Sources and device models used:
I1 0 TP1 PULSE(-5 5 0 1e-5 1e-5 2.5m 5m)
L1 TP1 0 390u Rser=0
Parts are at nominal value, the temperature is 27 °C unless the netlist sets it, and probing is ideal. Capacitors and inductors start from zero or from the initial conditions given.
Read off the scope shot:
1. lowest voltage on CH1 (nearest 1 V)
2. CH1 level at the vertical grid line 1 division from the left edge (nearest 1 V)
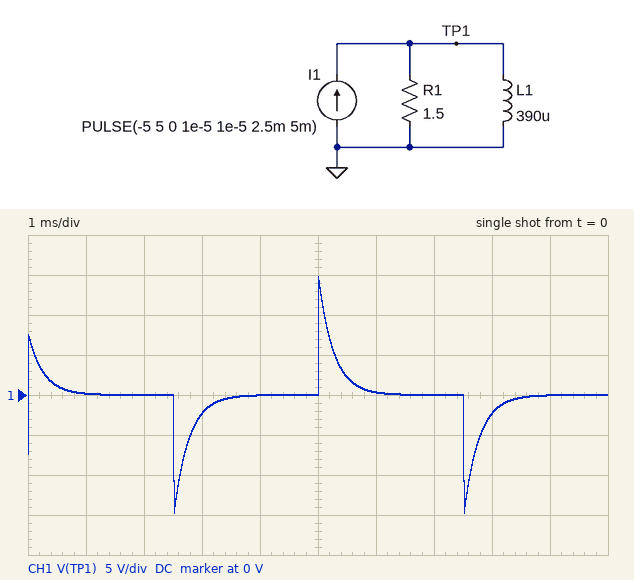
-15 V
0 V
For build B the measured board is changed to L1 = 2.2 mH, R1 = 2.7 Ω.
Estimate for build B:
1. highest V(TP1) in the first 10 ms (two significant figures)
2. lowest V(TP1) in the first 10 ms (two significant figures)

26 V
-26 V
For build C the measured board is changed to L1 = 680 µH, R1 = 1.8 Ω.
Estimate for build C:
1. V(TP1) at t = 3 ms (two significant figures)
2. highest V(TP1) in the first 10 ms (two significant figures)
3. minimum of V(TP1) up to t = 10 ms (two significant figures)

-5.0 V
18 V
-18 V
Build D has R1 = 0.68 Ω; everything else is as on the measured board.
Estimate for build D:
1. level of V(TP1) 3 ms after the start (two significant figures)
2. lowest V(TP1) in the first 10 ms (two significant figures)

-2.9 V
-6.7 V
